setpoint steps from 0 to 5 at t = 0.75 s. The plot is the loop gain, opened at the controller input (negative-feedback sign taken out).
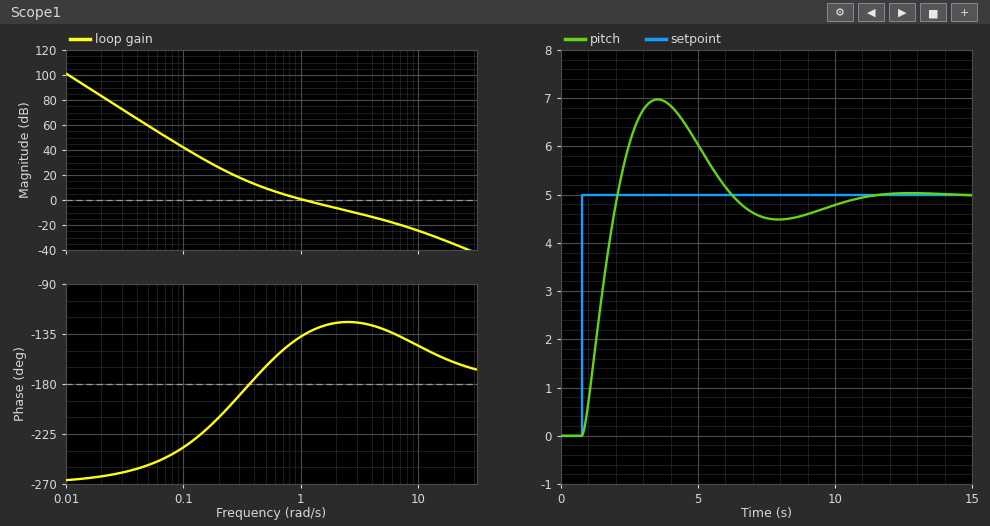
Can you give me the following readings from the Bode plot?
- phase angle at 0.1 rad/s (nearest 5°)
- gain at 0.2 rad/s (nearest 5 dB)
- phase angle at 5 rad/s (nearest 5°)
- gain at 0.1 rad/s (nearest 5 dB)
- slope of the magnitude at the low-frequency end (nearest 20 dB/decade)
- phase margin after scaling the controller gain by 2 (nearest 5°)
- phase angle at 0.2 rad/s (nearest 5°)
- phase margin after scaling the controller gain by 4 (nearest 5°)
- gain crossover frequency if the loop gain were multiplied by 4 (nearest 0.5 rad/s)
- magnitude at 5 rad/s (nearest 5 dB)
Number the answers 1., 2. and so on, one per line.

1. -235°
2. 25 dB
3. -130°
4. 40 dB
5. -60 dB/decade
6. 55°
7. -210°
8. 55°
9. 3.5 rad/s
10. -15 dB
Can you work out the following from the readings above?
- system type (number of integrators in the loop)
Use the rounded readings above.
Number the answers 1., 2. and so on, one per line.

1. 3
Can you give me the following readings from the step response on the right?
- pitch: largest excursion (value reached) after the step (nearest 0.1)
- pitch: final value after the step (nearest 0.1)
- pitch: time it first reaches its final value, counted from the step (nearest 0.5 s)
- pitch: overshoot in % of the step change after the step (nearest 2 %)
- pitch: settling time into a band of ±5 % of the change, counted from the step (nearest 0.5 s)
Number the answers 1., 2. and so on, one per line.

1. 7.0
2. 5.0
3. 1.5 s
4. 40 %
5. 9.0 s
